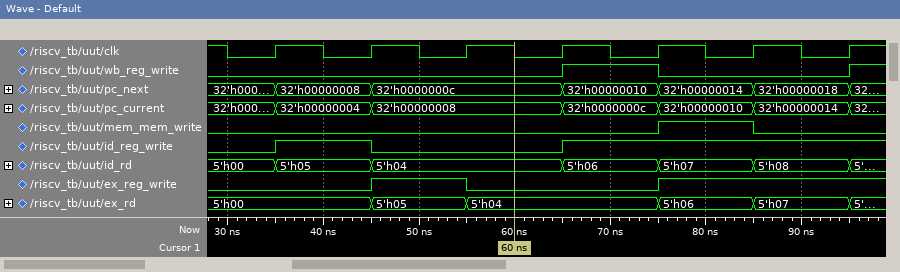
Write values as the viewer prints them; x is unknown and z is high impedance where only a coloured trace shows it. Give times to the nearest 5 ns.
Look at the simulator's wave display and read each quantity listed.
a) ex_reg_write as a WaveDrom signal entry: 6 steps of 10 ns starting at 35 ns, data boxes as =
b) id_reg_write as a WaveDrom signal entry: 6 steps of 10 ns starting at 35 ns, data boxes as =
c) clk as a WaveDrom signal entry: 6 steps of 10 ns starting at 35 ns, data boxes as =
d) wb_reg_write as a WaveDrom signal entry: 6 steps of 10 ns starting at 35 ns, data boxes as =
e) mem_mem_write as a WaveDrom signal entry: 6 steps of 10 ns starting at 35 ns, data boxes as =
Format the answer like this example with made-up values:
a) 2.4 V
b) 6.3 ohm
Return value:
a) {name: 'ex_reg_write', wave: '010.1.'}
b) {name: 'id_reg_write', wave: '10.1..'}
c) {name: 'clk', wave: 'p.....'}
d) {name: 'wb_reg_write', wave: '0..10.'}
e) {name: 'mem_mem_write', wave: '0...10'}
